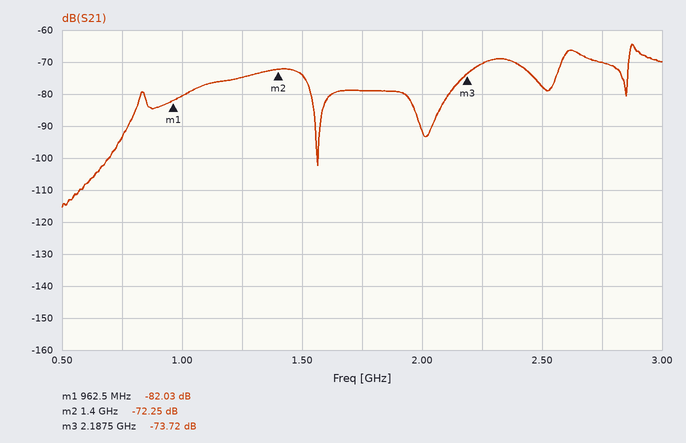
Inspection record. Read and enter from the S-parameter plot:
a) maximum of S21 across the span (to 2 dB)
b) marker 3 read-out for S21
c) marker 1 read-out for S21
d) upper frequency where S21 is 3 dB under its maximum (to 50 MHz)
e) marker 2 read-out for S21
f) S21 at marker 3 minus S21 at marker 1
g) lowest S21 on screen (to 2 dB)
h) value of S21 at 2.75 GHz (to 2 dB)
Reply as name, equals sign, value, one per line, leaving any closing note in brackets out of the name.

maximum of S21 across the span = -64 dB
marker 3 read-out for S21 = -73.72 dB
marker 1 read-out for S21 = -82.03 dB
upper frequency where S21 is 3 dB under its maximum = 2.90 GHz
marker 2 read-out for S21 = -72.25 dB
S21 at marker 3 minus S21 at marker 1 = 8.31 dB
lowest S21 on screen = -116 dB
value of S21 at 2.75 GHz = -70 dB
